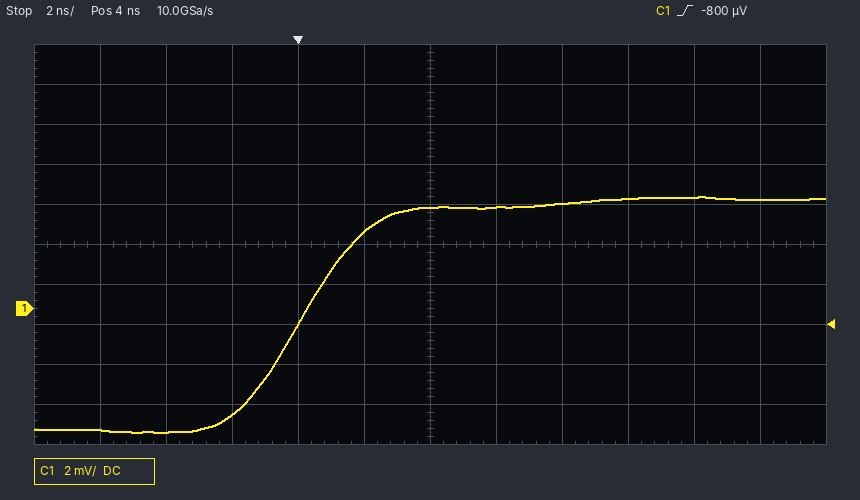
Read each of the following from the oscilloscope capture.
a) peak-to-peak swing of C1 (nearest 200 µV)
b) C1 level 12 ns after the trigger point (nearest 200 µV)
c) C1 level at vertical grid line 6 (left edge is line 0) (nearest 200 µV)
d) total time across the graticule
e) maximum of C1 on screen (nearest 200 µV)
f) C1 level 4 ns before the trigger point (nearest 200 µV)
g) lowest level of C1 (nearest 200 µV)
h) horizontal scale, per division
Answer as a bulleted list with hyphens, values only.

- 11.8 mV
- 5.6 mV
- 5.0 mV
- 24 ns
- 5.6 mV
- -6.2 mV
- -6.2 mV
- 2 ns
